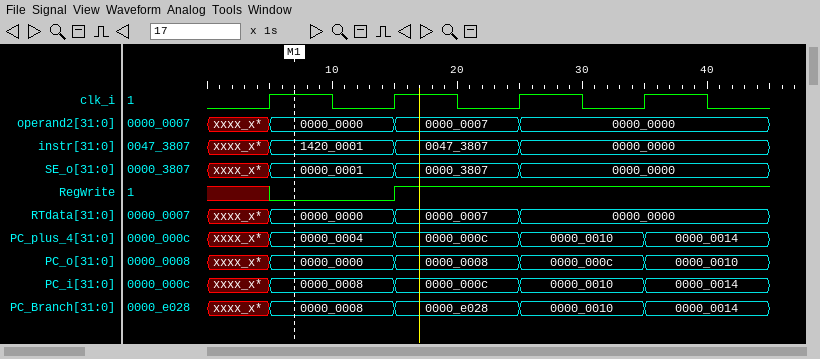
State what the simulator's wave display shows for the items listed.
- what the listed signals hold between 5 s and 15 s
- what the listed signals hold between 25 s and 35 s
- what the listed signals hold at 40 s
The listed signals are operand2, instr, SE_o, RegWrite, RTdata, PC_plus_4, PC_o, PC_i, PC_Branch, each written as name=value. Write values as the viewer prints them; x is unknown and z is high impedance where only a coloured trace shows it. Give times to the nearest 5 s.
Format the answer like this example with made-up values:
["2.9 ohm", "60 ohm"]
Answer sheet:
["operand2=0000_0000, instr=1420_0001, SE_o=0000_0001, RegWrite=0, RTdata=0000_0000, PC_plus_4=0000_0004, PC_o=0000_0000, PC_i=0000_0008, PC_Branch=0000_0008", "operand2=0000_0000, instr=0000_0000, SE_o=0000_0000, RegWrite=1, RTdata=0000_0000, PC_plus_4=0000_0010, PC_o=0000_000c, PC_i=0000_0010, PC_Branch=0000_0010", "operand2=0000_0000, instr=0000_0000, SE_o=0000_0000, RegWrite=1, RTdata=0000_0000, PC_plus_4=0000_0014, PC_o=0000_0010, PC_i=0000_0014, PC_Branch=0000_0014"]
